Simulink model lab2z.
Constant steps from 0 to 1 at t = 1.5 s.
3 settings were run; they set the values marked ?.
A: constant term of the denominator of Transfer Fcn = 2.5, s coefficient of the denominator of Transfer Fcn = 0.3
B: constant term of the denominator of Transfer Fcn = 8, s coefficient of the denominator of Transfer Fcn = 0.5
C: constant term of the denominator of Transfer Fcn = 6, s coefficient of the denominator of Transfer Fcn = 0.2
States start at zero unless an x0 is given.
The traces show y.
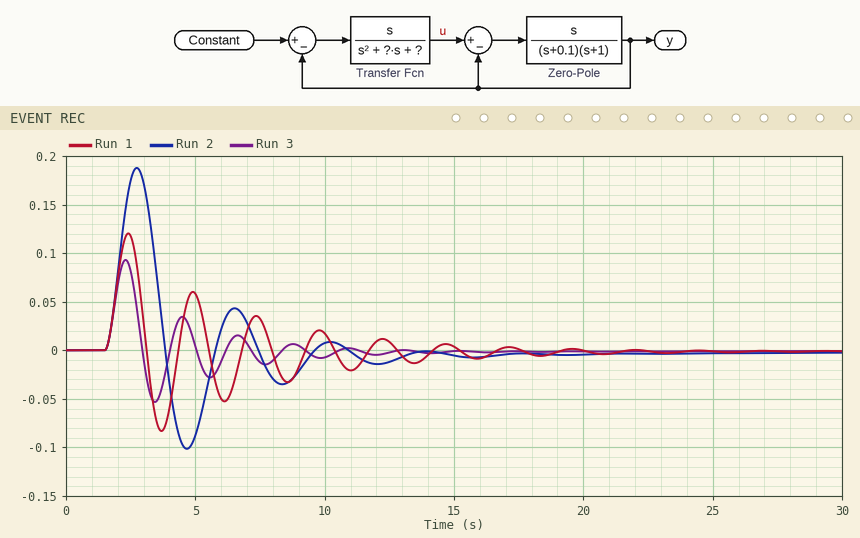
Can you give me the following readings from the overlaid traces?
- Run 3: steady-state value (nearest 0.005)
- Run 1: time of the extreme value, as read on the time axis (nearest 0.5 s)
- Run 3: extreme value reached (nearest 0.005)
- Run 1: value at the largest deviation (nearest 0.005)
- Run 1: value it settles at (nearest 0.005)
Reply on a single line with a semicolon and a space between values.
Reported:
0.000; 2.5 s; 0.095; 0.120; 0.000
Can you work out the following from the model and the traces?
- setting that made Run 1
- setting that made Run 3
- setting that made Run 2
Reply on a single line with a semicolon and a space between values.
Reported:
C; B; A
